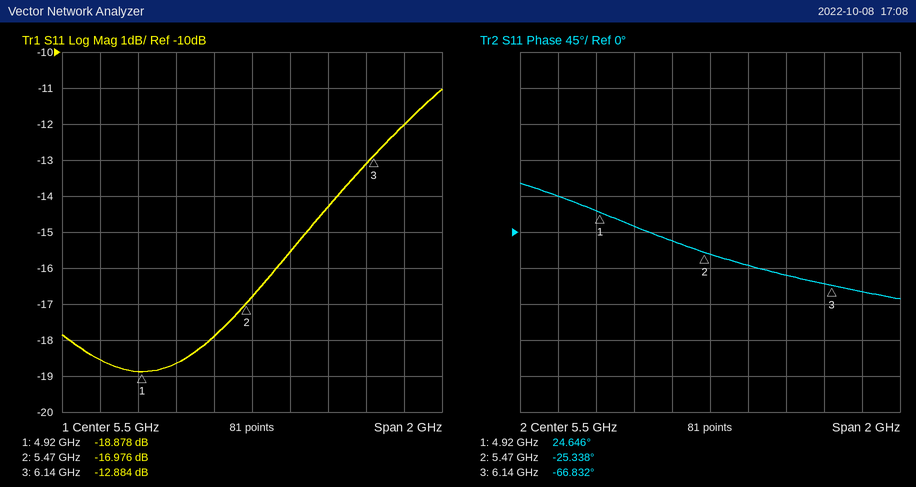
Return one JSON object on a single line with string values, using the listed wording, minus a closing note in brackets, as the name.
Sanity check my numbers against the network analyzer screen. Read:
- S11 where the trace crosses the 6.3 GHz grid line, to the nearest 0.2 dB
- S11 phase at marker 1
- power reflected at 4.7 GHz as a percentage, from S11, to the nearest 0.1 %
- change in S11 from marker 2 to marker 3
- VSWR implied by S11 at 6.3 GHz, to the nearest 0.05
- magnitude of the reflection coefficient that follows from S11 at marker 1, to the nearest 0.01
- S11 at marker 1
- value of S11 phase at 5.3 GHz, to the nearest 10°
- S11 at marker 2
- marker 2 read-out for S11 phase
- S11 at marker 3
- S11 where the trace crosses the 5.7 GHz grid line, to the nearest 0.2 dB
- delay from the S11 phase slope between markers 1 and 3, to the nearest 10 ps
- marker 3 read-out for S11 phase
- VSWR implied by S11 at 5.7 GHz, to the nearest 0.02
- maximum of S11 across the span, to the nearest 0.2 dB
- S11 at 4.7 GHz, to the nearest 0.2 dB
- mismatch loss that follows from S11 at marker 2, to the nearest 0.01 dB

{"S11 where the trace crosses the 6.3 GHz grid line, to the nearest 0.2 dB": "-12.0 dB", "S11 phase at marker 1": "24.646°", "power reflected at 4.7 GHz as a percentage, from S11, to the nearest 0.1 %": "1.4 %", "change in S11 from marker 2 to marker 3": "4.092 dB", "VSWR implied by S11 at 6.3 GHz, to the nearest 0.05": "1.65", "magnitude of the reflection coefficient that follows from S11 at marker 1, to the nearest 0.01": "0.11", "S11 at marker 1": "-18.878 dB", "value of S11 phase at 5.3 GHz, to the nearest 10°": "-10°", "S11 at marker 2": "-16.976 dB", "marker 2 read-out for S11 phase": "-25.338°", "S11 at marker 3": "-12.884 dB", "S11 where the trace crosses the 5.7 GHz grid line, to the nearest 0.2 dB": "-15.6 dB", "delay from the S11 phase slope between markers 1 and 3, to the nearest 10 ps": "210 ps", "marker 3 read-out for S11 phase": "-66.832°", "VSWR implied by S11 at 5.7 GHz, to the nearest 0.02": "1.40", "maximum of S11 across the span, to the nearest 0.2 dB": "-11.0 dB", "S11 at 4.7 GHz, to the nearest 0.2 dB": "-18.6 dB", "mismatch loss that follows from S11 at marker 2, to the nearest 0.01 dB": "0.09 dB"}
